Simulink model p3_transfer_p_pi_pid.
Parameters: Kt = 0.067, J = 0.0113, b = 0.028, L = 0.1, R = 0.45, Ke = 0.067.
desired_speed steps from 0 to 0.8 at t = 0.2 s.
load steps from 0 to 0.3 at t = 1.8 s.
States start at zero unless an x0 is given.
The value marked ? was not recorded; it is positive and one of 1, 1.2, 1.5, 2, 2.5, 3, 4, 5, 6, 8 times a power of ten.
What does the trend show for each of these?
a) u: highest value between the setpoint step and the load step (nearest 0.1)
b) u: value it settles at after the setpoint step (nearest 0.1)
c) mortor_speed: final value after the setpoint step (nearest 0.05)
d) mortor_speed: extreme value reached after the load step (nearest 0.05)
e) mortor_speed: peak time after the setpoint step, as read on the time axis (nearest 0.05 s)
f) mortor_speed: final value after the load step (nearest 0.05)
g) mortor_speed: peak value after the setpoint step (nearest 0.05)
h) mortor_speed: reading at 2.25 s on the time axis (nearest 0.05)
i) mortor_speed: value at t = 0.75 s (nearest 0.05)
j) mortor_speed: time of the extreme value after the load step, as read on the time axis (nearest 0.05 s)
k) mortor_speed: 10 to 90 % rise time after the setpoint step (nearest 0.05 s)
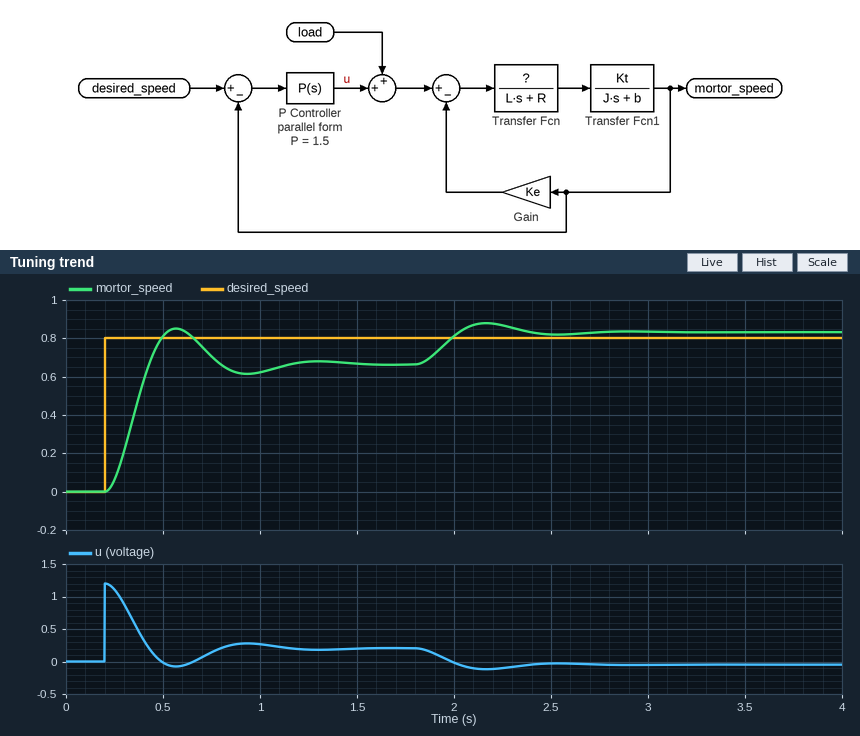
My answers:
1.2
0.2
0.65
0.90
0.55 s
0.85
0.85
0.85
0.70
2.15 s
0.15 s
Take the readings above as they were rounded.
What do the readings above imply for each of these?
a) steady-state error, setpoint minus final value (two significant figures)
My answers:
0.15
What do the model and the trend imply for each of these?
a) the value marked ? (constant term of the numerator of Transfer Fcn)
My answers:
0.8
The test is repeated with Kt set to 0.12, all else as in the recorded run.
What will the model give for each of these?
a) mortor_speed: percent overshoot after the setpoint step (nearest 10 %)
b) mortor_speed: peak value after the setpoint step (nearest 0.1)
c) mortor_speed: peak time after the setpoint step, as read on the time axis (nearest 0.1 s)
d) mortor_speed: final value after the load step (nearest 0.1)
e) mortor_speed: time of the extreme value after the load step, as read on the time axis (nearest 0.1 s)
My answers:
40 %
1.0
0.5 s
0.9
2.1 s
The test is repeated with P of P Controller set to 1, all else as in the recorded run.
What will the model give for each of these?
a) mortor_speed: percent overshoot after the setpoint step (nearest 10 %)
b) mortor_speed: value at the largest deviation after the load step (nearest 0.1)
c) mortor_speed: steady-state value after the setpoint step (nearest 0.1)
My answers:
20 %
0.9
0.6
